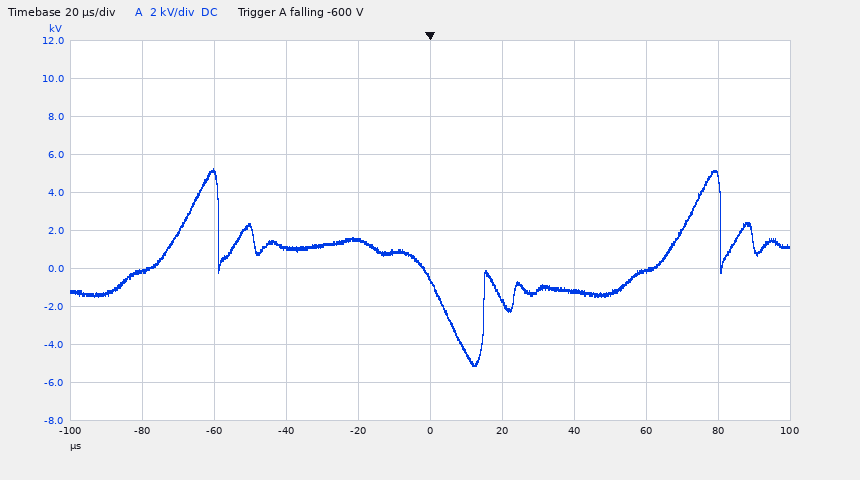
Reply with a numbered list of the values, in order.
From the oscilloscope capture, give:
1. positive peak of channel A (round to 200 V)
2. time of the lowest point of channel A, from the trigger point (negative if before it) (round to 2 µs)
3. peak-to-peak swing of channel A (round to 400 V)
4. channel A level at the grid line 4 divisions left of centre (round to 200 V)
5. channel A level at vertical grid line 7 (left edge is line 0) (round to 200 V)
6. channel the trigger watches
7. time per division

1. 5.2 kV
2. +12 µs
3. 10.4 kV
4. -200 V
5. -1.2 kV
6. channel A
7. 20 µs
